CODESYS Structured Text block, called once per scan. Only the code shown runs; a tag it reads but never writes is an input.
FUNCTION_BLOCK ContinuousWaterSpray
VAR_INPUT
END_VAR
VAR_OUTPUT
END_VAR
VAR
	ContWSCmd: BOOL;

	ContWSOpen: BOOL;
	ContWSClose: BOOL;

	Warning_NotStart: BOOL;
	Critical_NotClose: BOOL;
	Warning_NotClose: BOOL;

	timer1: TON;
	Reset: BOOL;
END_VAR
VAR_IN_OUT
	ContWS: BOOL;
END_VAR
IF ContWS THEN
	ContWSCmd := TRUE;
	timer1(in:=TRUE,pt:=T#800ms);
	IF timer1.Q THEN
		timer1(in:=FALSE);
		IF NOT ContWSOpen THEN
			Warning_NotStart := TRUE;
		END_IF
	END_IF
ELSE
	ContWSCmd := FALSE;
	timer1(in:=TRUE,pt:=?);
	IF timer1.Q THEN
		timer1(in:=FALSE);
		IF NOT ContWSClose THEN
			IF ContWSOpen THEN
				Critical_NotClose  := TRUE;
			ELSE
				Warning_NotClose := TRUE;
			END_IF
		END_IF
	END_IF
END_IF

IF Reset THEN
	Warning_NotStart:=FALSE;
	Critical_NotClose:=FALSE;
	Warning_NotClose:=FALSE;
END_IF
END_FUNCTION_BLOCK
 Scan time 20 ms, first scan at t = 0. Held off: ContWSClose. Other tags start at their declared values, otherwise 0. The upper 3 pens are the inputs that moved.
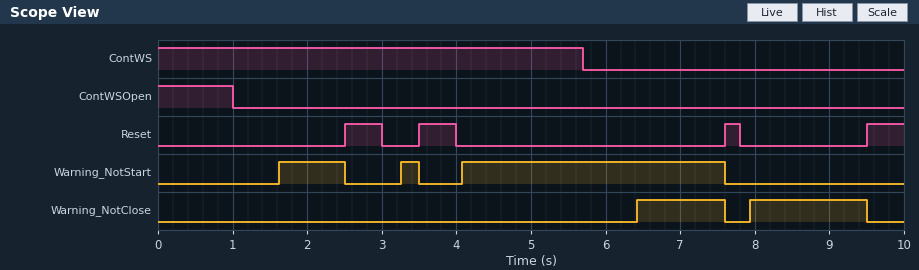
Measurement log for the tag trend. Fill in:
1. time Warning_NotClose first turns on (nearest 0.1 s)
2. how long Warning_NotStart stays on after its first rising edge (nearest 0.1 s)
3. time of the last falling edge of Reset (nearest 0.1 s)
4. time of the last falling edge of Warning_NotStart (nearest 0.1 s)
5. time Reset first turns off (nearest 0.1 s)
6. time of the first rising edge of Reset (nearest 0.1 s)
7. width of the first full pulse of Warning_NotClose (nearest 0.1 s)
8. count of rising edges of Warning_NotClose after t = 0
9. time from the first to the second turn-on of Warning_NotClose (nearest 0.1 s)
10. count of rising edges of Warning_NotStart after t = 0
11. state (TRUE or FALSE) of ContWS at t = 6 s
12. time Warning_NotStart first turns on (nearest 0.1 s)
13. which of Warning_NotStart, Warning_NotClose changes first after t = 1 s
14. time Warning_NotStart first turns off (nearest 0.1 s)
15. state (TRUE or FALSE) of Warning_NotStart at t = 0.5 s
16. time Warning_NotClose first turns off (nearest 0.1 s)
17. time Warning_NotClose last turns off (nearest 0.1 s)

6.4 s
0.9 s
7.8 s
7.6 s
3.0 s
2.5 s
1.2 s
2
1.5 s
3
FALSE
1.6 s
Warning_NotStart
2.5 s
FALSE
7.6 s
9.5 s
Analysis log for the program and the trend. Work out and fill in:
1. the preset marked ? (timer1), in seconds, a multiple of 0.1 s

1.5 s
